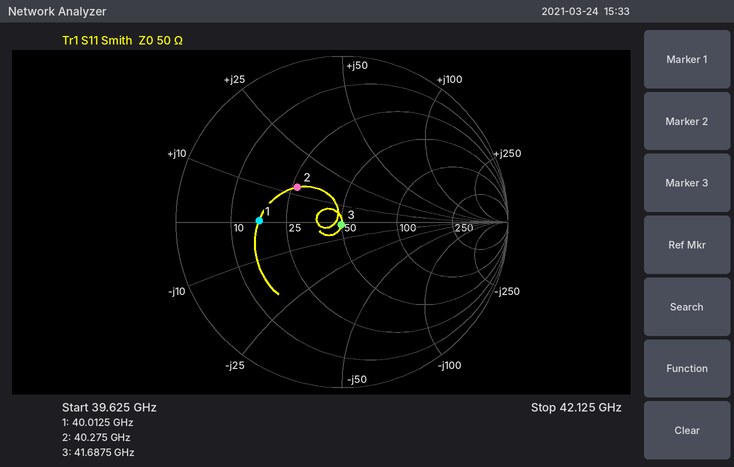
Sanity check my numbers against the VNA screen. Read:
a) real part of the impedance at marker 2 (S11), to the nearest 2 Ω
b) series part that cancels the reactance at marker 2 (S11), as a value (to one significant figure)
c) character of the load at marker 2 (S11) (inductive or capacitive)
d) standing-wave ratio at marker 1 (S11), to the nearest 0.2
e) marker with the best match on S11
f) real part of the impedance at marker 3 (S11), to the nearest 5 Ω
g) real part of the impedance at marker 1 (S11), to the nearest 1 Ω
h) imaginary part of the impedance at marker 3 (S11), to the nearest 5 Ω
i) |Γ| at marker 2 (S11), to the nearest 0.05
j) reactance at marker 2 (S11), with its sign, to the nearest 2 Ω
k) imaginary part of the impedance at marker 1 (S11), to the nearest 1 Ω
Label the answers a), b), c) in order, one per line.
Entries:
a) 26 Ω
b) 300 fF
c) inductive
d) 3.0
e) marker 3
f) 50 Ω
g) 17 Ω
h) 0 Ω
i) 0.35
j) +12 Ω
k) 0 Ω
